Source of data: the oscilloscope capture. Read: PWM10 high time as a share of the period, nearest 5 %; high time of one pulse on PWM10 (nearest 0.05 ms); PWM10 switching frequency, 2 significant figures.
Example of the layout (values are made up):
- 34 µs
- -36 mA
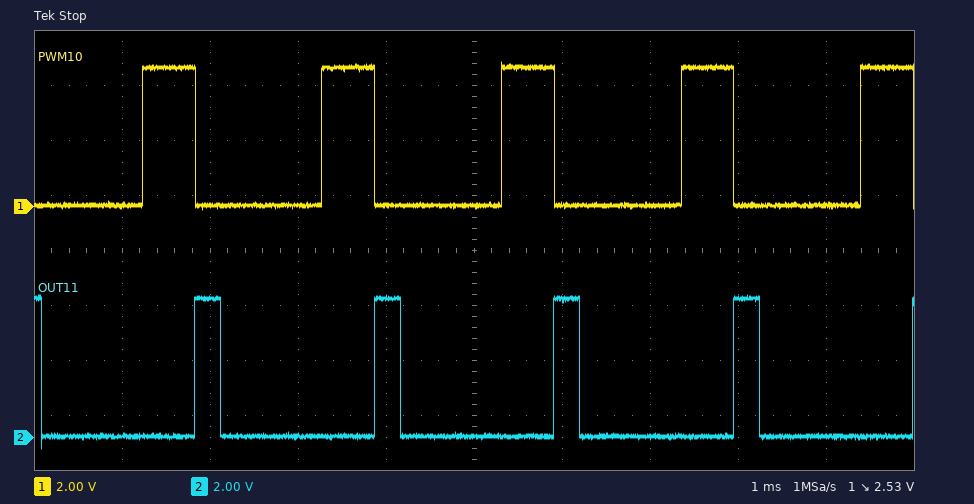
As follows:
- 30 %
- 0.60 ms
- 490 Hz
